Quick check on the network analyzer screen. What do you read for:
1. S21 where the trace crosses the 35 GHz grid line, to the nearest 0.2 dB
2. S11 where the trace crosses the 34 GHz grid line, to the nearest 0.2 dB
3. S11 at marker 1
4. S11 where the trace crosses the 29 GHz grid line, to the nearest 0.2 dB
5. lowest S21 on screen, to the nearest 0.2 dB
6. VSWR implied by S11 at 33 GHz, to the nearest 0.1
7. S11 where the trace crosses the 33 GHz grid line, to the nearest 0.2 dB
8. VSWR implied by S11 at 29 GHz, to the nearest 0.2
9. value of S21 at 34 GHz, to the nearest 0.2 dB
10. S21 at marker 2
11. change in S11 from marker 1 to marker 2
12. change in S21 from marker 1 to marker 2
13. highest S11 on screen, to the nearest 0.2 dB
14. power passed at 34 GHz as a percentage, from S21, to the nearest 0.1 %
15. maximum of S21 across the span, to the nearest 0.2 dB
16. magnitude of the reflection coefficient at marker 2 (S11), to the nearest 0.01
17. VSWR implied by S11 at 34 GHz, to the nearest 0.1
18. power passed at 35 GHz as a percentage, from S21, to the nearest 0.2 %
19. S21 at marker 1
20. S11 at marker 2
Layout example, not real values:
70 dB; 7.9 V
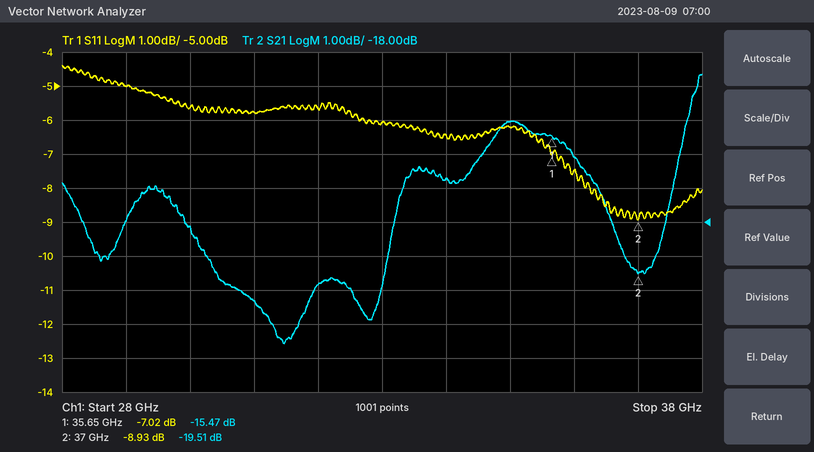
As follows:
-15.0 dB; -6.4 dB; -7.02 dB; -5.0 dB; -21.6 dB; 3.0; -6.0 dB; 3.6; -16.8 dB; -19.51 dB; -1.91 dB; -4.04 dB; -4.4 dB; 2.1 %; -13.6 dB; 0.36; 2.8; 3.2 %; -15.47 dB; -8.93 dB
